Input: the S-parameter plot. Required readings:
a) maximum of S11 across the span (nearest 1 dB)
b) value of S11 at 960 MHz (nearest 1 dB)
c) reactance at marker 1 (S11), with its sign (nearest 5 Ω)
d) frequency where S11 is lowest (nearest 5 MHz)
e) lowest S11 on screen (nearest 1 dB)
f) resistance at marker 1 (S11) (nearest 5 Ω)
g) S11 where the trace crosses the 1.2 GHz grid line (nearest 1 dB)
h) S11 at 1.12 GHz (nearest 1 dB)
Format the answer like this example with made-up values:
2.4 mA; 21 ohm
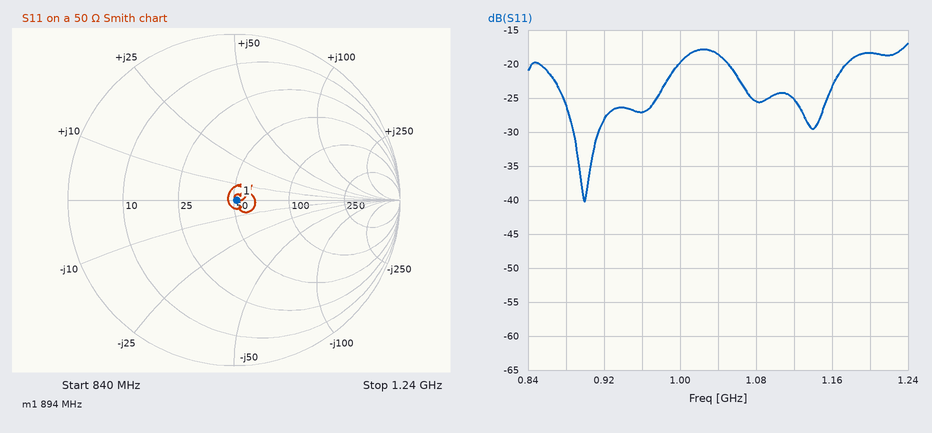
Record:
-17 dB; -27 dB; 0 Ω; 900 MHz; -40 dB; 50 Ω; -18 dB; -25 dB
